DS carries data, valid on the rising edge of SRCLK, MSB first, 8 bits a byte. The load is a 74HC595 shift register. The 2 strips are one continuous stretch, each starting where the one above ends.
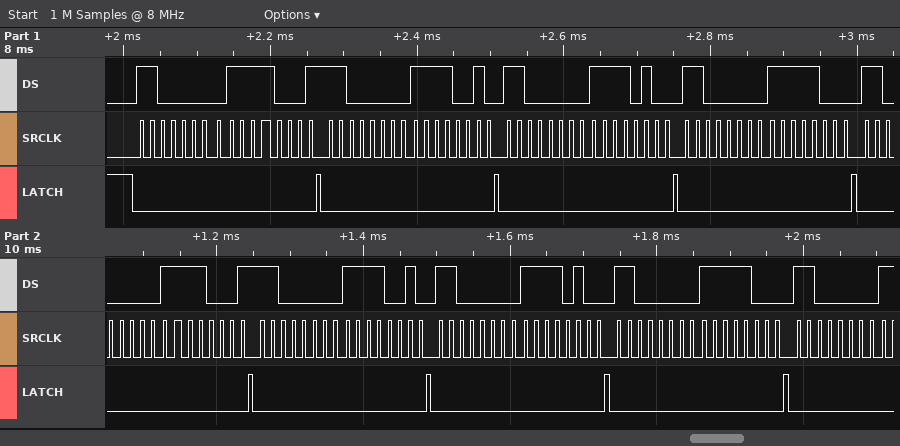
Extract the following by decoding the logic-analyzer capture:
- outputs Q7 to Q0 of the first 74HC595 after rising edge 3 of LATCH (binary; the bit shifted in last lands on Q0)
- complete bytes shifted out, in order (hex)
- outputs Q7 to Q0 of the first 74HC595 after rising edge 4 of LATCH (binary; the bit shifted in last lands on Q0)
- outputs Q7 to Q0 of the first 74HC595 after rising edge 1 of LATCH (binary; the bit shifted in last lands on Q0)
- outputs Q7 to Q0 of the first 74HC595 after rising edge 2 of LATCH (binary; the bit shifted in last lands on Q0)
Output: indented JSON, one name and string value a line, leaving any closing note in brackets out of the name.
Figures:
{
  "outputs Q7 to Q0 of the first 74HC595 after rising edge 3 of LATCH": "11110100",
  "complete bytes shifted out, in order": "C0 F1 C0 F2 C0 F4 C0 F8 C0 F1 C0 F2 C0 F4 C0 F8 C0",
  "outputs Q7 to Q0 of the first 74HC595 after rising edge 4 of LATCH": "11111000",
  "outputs Q7 to Q0 of the first 74HC595 after rising edge 1 of LATCH": "11110001",
  "outputs Q7 to Q0 of the first 74HC595 after rising edge 2 of LATCH": "11110010"
}
